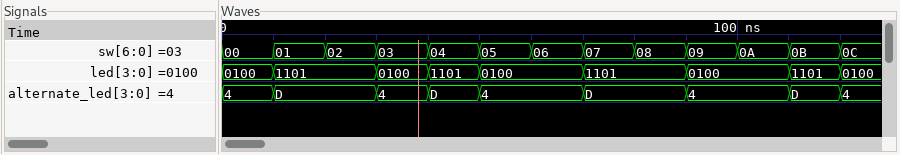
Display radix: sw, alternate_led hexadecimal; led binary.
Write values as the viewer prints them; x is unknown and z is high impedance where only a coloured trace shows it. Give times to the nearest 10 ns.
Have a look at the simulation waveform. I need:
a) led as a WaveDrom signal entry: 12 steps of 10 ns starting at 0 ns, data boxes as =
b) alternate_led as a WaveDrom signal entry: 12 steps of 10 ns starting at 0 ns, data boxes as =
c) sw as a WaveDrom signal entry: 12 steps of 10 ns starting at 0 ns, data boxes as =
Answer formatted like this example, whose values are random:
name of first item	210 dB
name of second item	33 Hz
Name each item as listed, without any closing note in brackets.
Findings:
led as a WaveDrom signal entry: 12 steps of 10 ns starting at 0 ns, data boxes as =	{name: 'led', wave: '==.===.=.=.=', data: '0100 1101 0100 1101 0100 1101 0100 1101'}
alternate_led as a WaveDrom signal entry: 12 steps of 10 ns starting at 0 ns, data boxes as =	{name: 'alternate_led', wave: '==.===.=.=.=', data: '4 D 4 D 4 D 4 D'}
sw as a WaveDrom signal entry: 12 steps of 10 ns starting at 0 ns, data boxes as =	{name: 'sw', wave: '============', data: '00 01 02 03 04 05 06 07 08 09 0A 0B'}
